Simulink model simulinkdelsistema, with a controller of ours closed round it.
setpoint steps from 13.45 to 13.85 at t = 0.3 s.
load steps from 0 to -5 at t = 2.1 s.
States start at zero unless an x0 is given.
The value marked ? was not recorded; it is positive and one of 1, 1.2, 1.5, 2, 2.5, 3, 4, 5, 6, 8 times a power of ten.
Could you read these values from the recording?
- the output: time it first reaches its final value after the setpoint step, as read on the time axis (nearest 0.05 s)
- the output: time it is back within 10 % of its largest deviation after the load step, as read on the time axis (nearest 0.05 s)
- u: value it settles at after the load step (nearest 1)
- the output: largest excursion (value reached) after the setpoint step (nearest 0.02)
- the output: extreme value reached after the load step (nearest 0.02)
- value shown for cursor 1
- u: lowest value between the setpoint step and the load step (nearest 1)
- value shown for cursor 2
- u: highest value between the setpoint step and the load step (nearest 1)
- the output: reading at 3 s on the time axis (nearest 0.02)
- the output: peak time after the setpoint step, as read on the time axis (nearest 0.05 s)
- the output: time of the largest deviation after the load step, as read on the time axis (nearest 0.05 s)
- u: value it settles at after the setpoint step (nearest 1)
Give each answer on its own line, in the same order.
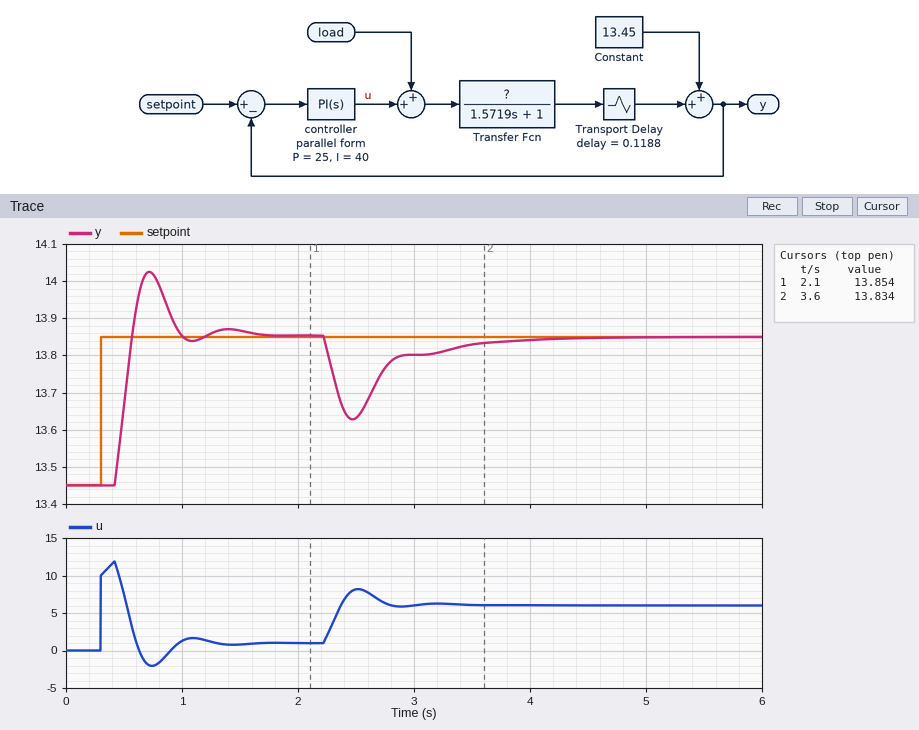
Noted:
0.55 s
3.45 s
6
14.02
13.62
13.854
-2
13.834
12
13.80
0.70 s
2.45 s
1
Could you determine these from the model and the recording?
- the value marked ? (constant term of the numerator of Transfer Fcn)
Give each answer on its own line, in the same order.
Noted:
0.4
